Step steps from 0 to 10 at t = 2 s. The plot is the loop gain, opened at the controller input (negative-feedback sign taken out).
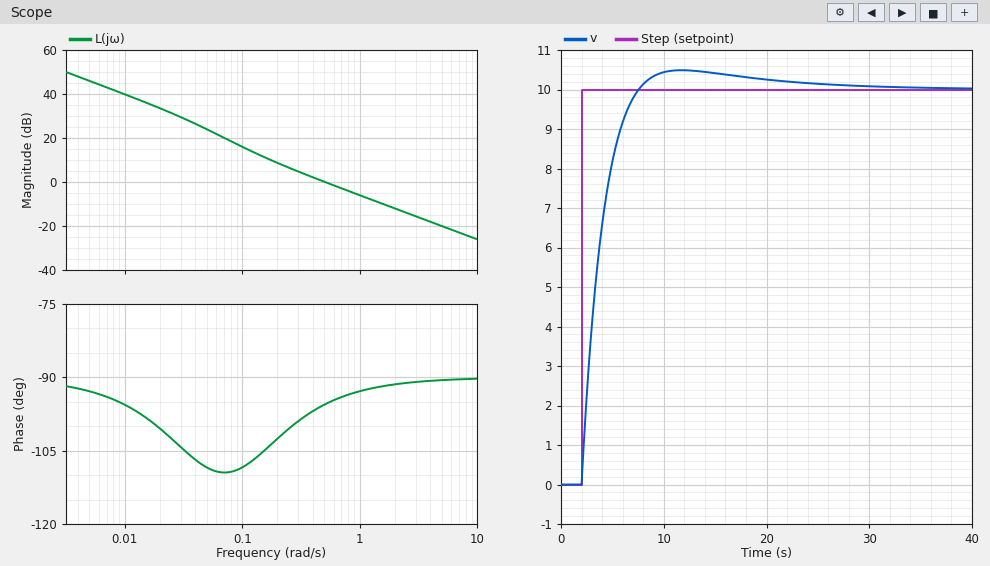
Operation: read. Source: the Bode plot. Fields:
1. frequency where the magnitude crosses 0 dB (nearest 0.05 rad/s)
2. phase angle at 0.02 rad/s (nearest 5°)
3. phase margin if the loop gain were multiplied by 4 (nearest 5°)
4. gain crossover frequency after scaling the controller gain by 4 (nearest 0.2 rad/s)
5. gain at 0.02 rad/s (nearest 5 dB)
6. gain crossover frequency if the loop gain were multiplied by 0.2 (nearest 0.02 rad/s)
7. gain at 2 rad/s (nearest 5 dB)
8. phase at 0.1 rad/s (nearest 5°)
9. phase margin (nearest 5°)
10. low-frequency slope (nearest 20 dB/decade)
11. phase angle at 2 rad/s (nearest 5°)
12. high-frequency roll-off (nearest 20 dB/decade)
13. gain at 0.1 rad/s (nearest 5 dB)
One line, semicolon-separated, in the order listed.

0.50 rad/s; -100°; 90°; 2.0 rad/s; 35 dB; 0.12 rad/s; -10 dB; -110°; 85°; -20 dB/decade; -90°; -20 dB/decade; 15 dB
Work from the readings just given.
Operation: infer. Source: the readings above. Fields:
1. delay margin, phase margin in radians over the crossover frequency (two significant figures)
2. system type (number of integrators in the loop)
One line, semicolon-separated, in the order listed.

3.0 s; 1
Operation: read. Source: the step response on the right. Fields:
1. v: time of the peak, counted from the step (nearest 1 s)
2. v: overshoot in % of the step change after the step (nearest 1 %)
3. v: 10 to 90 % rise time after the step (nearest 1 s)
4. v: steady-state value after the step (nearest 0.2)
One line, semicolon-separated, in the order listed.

10 s; 5 %; 4 s; 10.0
